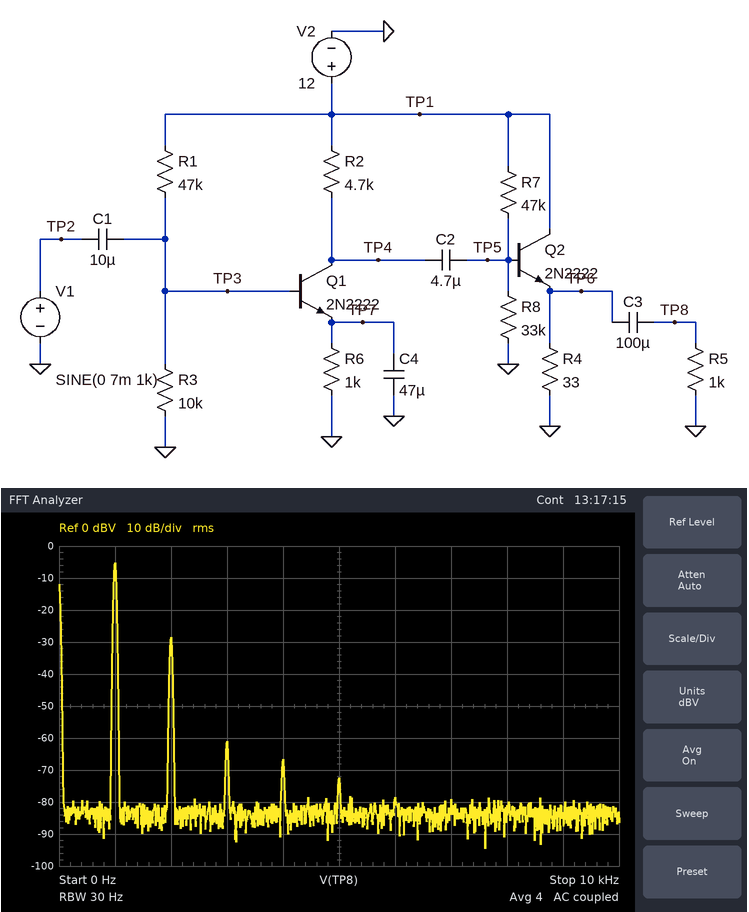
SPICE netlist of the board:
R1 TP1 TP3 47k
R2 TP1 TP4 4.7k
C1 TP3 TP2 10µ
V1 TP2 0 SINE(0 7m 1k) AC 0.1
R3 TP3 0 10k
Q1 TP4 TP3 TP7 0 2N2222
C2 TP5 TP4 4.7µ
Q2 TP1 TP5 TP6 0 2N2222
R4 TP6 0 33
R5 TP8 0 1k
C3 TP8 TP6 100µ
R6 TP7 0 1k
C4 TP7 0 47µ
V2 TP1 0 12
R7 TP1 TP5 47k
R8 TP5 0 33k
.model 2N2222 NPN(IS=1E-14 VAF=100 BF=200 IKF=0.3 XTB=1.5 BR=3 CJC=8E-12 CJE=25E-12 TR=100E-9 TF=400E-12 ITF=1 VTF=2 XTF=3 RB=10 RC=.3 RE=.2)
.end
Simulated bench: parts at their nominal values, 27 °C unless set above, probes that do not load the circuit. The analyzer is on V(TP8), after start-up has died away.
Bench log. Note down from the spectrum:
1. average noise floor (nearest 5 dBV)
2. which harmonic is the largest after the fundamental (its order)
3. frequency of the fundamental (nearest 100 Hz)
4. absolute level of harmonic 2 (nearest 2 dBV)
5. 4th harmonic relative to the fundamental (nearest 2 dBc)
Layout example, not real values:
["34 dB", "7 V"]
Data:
["-85 dBV", "2", "1.0 kHz", "-28 dBV", "-62 dBc"]
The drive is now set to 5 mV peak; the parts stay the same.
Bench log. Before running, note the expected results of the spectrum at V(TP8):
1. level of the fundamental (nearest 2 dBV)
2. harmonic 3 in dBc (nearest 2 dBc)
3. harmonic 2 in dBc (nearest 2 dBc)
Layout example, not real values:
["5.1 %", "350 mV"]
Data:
["-8 dBV", "-58 dBc", "-26 dBc"]
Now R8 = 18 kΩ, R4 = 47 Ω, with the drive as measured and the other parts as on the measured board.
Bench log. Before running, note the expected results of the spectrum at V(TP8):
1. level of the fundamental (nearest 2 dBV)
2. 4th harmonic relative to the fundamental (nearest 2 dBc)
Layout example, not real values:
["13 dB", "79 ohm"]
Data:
["-4 dBV", "-58 dBc"]
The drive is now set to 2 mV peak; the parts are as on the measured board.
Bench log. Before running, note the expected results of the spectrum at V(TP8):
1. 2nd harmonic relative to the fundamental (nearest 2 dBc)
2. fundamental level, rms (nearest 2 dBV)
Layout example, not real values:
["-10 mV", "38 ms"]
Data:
["-34 dBc", "-16 dBV"]
